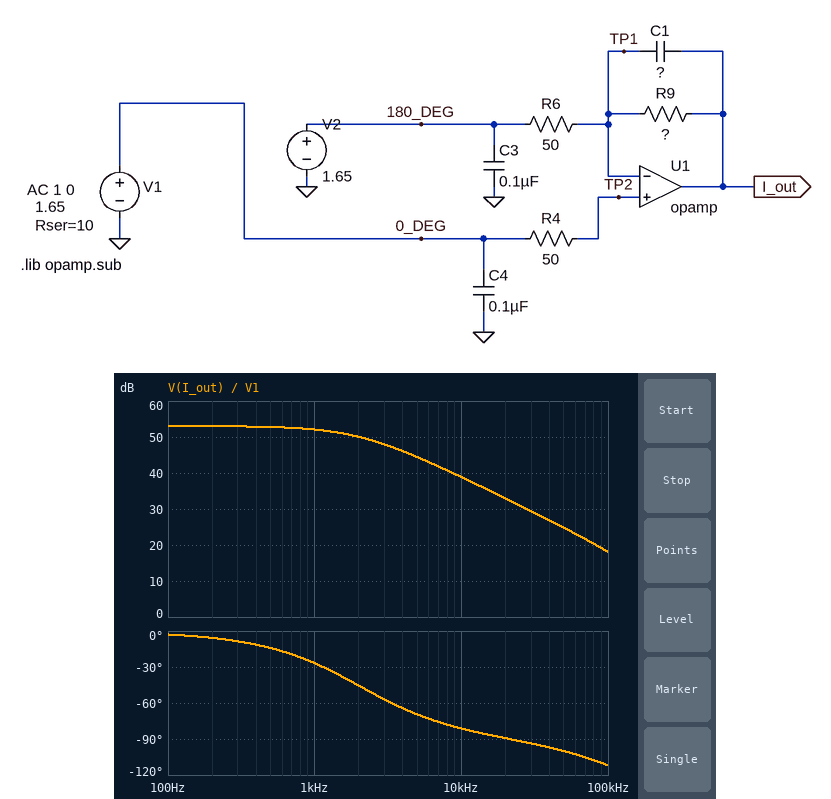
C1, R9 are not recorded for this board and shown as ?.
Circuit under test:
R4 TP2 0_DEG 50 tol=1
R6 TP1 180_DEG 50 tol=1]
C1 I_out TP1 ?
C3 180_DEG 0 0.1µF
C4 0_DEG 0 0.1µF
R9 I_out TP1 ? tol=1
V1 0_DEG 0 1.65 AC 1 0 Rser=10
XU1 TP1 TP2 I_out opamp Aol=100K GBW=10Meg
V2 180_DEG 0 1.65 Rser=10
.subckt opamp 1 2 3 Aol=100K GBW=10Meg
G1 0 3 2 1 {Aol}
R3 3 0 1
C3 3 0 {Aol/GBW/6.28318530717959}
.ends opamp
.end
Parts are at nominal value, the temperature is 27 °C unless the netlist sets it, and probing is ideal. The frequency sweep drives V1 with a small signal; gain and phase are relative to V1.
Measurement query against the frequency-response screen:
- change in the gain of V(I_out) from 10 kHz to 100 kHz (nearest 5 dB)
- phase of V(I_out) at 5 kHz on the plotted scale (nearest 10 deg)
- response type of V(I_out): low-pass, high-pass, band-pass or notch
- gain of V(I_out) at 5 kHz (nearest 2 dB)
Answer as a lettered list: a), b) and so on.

a) -20 dB
b) -70 deg
c) low-pass
d) 44 dB
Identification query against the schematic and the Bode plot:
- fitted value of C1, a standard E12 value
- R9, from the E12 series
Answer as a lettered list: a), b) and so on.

a) 2.7 nF
b) 27 kΩ
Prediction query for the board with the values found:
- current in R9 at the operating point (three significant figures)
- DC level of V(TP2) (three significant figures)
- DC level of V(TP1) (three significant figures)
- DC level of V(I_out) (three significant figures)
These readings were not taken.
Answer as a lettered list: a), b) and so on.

a) 274 nA
b) 1.65 V
c) 1.65 V
d) 1.64 V
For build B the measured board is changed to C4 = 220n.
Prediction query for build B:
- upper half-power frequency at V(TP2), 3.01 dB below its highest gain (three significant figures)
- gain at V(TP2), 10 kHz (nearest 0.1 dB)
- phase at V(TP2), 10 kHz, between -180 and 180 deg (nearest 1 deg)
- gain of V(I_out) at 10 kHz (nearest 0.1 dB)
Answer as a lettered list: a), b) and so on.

a) 72.3 kHz
b) -0.1 dB
c) -8 deg
d) 38.8 dB
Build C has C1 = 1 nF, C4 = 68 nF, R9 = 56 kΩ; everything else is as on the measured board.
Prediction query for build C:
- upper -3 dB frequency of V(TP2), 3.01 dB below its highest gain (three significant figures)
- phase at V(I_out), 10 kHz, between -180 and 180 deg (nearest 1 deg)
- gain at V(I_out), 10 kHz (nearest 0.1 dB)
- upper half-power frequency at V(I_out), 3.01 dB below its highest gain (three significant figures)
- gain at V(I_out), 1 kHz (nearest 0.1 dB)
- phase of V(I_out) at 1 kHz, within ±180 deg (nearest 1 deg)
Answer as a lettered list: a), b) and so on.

a) 234 kHz
b) -79 deg
c) 46.2 dB
d) 2.27 kHz
e) 58.6 dB
f) -24 deg
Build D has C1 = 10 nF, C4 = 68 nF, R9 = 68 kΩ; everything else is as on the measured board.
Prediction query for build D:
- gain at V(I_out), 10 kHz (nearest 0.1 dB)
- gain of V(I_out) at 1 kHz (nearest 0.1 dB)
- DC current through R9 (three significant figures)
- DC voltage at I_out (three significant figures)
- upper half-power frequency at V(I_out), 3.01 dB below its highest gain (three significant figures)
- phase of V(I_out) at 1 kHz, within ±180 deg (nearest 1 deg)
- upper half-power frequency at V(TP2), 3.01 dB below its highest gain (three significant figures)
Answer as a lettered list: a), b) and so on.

a) 28.3 dB
b) 48.0 dB
c) 272 nA
d) 1.63 V
e) 231 Hz
f) -77 deg
g) 234 kHz
